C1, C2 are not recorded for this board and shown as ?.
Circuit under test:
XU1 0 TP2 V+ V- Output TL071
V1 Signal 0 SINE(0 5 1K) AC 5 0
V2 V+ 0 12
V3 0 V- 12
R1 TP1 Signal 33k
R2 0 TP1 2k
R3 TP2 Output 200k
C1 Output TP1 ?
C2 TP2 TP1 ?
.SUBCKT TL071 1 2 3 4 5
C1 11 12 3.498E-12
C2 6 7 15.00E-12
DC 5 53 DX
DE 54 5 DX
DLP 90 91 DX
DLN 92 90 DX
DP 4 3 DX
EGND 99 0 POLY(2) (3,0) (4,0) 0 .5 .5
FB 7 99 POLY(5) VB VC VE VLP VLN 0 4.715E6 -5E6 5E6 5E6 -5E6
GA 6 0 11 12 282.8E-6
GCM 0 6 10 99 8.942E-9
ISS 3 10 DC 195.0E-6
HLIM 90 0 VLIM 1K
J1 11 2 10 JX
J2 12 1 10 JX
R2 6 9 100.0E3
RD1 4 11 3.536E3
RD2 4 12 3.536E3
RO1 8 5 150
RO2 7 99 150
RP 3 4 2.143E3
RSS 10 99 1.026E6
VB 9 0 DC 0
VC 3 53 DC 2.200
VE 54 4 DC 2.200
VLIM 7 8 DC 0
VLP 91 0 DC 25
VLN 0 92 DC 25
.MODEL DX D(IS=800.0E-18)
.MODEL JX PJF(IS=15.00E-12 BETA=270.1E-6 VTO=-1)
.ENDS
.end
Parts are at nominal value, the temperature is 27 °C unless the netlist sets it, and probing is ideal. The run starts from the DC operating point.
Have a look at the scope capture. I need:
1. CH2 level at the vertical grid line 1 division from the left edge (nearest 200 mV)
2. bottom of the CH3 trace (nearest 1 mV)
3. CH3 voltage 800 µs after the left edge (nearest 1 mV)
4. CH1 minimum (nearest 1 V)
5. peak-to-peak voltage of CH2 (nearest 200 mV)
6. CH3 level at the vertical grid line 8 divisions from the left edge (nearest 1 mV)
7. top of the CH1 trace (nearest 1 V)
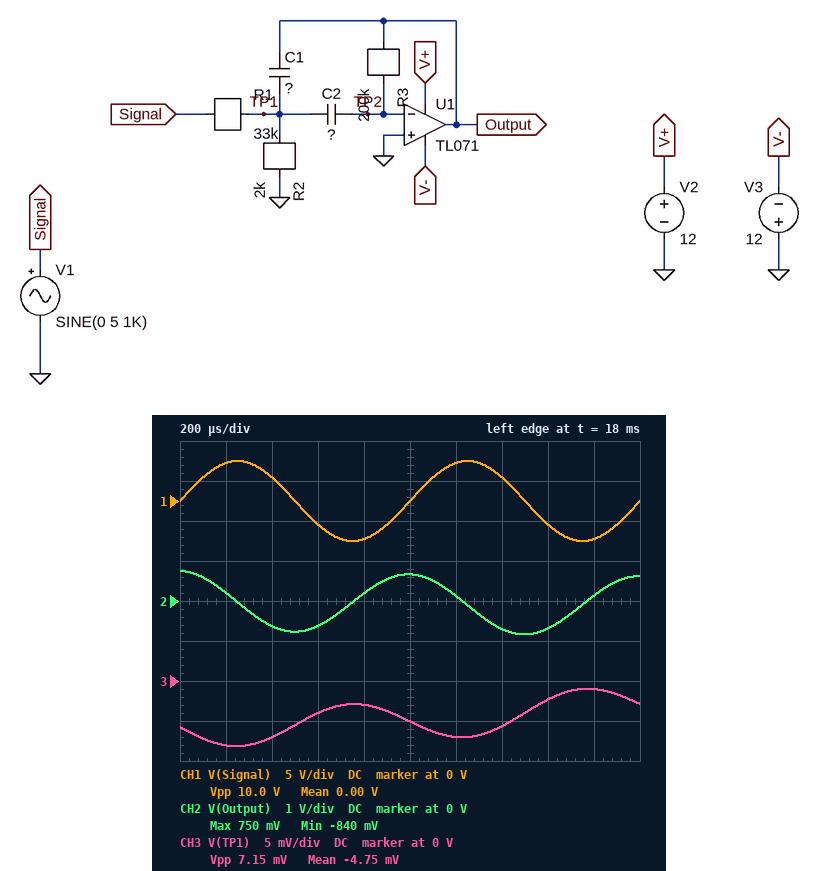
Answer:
200 mV
-8 mV
-3 mV
-5 V
1.6 V
-2 mV
5 V
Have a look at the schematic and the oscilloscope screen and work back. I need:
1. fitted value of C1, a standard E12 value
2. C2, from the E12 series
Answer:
33 nF
220 nF
